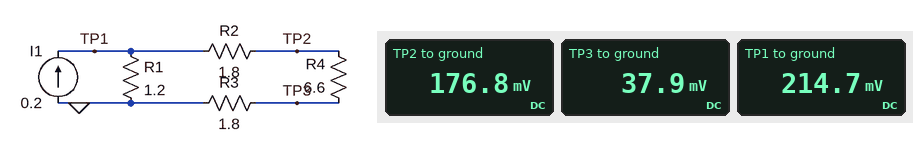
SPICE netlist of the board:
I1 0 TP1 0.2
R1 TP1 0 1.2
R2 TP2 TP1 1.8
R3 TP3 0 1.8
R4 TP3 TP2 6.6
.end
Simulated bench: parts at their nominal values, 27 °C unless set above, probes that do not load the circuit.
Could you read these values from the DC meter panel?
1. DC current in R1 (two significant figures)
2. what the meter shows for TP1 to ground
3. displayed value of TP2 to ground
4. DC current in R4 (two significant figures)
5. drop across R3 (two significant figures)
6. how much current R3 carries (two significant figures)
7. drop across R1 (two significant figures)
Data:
180 mA
214.7 mV
176.8 mV
21 mA
38 mV
21 mA
210 mV
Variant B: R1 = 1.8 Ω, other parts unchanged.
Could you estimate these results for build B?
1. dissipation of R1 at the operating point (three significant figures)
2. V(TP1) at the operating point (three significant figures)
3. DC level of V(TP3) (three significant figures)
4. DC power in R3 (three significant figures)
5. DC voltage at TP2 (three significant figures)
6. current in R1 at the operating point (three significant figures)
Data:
52.0 mW
306 mV
54.0 mV
1.62 mW
252 mV
170 mA
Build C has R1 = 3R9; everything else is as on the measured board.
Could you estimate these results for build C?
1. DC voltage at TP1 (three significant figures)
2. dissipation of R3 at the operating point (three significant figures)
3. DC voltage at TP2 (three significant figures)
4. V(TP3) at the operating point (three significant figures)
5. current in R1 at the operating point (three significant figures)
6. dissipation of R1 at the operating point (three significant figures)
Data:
564 mV
5.51 mW
465 mV
99.6 mV
145 mA
81.6 mW
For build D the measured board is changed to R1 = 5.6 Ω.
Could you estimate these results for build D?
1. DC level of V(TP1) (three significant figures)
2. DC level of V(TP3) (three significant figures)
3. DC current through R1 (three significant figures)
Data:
723 mV
128 mV
129 mA
